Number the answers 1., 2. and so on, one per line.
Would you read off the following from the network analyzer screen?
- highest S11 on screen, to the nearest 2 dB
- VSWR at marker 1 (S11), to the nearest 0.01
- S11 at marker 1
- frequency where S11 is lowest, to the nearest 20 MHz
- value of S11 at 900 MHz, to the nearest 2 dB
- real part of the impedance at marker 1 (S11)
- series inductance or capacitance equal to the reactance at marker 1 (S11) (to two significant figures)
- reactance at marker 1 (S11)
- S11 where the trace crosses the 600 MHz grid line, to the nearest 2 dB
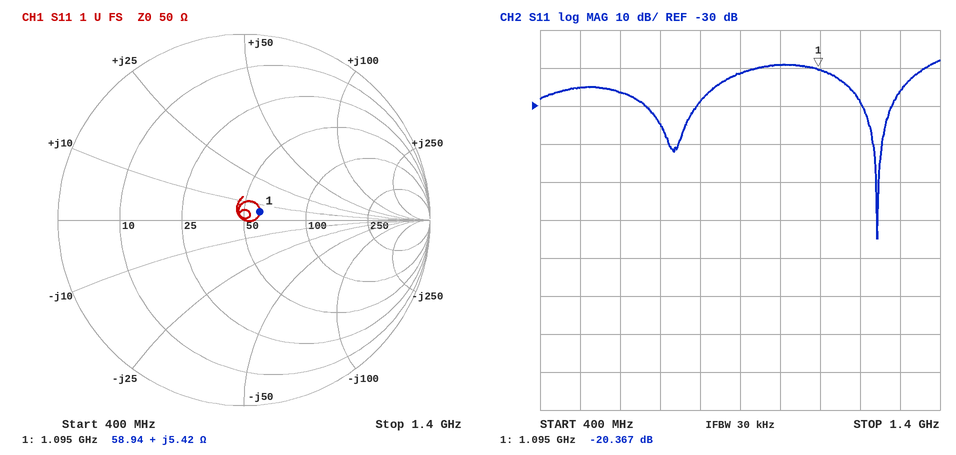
1. -18 dB
2. 1.21
3. -20.367 dB
4. 1.24 GHz
5. -22 dB
6. 58.94 Ω
7. 790 pH
8. +5.42 Ω
9. -26 dB
